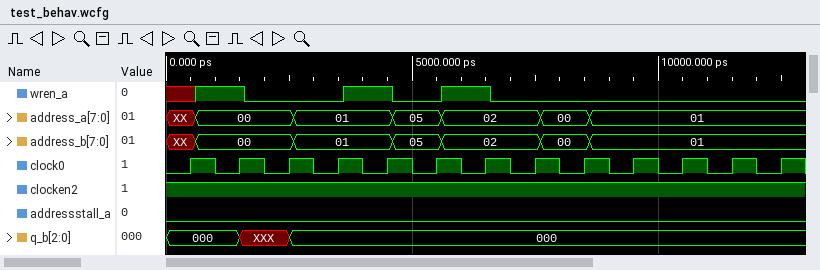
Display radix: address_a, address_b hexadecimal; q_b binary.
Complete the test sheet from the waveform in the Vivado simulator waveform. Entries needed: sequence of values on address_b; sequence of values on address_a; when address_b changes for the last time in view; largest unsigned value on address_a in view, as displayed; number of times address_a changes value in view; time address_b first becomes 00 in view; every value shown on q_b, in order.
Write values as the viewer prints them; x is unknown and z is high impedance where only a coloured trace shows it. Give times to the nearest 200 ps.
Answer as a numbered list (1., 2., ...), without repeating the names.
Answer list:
1. XX, 00, 01, 05, 02, 00, 01
2. XX, 00, 01, 05, 02, 00, 01
3. 8600 ps
4. 05
5. 6
6. 600 ps
7. 000, XXX, 000
